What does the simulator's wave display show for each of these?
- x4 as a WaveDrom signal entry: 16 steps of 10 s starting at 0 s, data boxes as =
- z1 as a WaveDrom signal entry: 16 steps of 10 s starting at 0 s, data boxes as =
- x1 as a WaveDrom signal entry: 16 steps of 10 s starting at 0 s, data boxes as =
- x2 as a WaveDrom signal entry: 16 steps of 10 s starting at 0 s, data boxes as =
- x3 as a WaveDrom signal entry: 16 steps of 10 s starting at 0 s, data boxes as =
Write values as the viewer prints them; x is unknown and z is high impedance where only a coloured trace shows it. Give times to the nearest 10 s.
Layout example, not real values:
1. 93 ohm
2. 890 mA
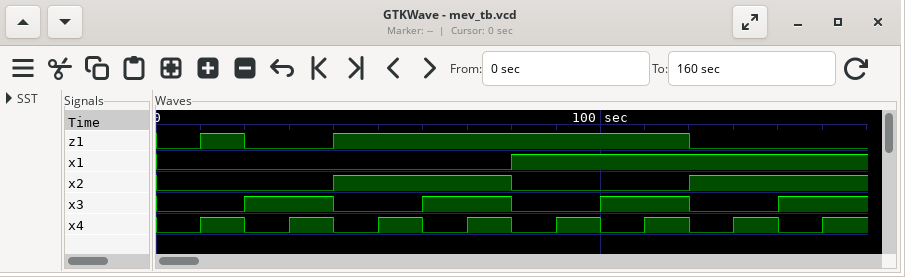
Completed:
1. {name: 'x4', wave: '0101010101010101'}
2. {name: 'z1', wave: '010.1.......0...'}
3. {name: 'x1', wave: '0.......1.......'}
4. {name: 'x2', wave: '0...1...0...1...'}
5. {name: 'x3', wave: '0.1.0.1.0.1.0.1.'}
